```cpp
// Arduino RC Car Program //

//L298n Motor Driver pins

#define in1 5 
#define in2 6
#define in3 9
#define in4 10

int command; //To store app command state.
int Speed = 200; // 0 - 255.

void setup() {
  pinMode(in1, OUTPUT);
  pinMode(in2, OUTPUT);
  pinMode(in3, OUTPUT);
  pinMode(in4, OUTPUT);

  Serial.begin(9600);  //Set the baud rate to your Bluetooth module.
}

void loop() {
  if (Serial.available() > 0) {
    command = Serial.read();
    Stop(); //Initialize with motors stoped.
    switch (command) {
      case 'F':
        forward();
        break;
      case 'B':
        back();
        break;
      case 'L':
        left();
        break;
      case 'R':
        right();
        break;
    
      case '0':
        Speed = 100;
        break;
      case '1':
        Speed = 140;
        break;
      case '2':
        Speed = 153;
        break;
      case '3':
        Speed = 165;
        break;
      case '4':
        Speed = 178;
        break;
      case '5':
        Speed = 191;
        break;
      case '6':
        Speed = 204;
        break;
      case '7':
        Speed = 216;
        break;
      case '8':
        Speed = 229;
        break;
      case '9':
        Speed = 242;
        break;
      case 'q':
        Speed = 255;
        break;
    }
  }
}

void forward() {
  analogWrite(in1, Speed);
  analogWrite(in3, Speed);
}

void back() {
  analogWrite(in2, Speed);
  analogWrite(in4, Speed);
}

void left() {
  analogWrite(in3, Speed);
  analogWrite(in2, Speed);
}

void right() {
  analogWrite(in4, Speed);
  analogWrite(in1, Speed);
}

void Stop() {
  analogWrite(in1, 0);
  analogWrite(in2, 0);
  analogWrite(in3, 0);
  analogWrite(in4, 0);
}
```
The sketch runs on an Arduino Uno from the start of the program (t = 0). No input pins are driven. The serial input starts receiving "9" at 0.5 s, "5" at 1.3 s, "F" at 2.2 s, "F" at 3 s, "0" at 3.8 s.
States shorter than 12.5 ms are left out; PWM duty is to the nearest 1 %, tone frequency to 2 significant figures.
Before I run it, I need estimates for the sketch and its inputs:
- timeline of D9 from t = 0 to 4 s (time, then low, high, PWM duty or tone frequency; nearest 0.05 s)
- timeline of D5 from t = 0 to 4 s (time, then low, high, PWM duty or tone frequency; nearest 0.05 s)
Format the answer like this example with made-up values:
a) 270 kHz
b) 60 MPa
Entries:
a) 0 s low; 2.2 s PWM 75 %; 3.8 s low
b) 0 s low; 2.2 s PWM 75 %; 3.8 s low
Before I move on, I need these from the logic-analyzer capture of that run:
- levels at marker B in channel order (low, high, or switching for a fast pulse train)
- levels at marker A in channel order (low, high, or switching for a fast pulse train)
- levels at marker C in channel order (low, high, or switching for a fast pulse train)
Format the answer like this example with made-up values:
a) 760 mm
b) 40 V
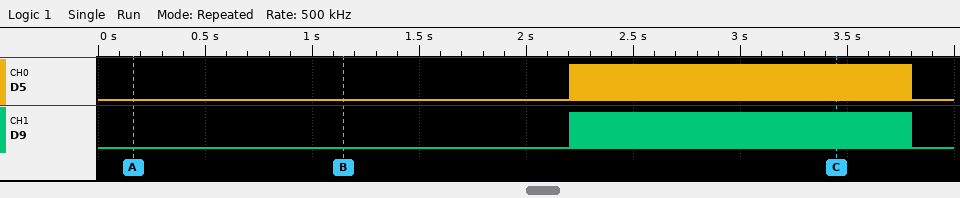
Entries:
a) D5 low, D9 low
b) D5 low, D9 low
c) D5 switching, D9 switching
